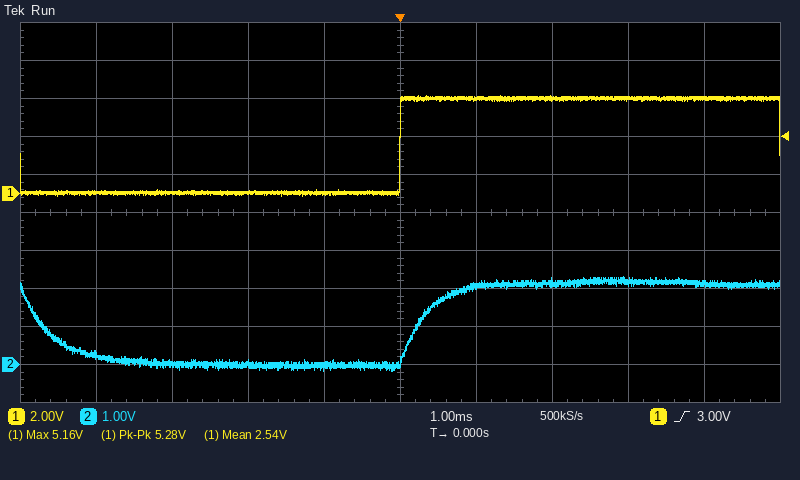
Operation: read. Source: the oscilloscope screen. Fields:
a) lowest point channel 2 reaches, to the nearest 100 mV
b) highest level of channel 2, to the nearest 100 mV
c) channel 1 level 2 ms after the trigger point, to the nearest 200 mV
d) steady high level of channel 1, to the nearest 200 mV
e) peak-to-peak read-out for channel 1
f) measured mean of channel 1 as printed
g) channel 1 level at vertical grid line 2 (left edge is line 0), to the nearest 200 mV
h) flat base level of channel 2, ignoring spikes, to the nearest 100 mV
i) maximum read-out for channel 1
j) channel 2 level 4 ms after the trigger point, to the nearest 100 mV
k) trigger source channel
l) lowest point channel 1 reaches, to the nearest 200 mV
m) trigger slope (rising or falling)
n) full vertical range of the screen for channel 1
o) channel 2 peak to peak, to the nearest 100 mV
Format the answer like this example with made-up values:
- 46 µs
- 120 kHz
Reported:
- -200 mV
- 2.3 V
- 5.0 V
- 5.0 V
- 5.28 V
- 2.54 V
- 0.0 V
- 0.0 V
- 5.16 V
- 2.1 V
- channel 1
- -200 mV
- rising
- 20 V
- 2.5 V
